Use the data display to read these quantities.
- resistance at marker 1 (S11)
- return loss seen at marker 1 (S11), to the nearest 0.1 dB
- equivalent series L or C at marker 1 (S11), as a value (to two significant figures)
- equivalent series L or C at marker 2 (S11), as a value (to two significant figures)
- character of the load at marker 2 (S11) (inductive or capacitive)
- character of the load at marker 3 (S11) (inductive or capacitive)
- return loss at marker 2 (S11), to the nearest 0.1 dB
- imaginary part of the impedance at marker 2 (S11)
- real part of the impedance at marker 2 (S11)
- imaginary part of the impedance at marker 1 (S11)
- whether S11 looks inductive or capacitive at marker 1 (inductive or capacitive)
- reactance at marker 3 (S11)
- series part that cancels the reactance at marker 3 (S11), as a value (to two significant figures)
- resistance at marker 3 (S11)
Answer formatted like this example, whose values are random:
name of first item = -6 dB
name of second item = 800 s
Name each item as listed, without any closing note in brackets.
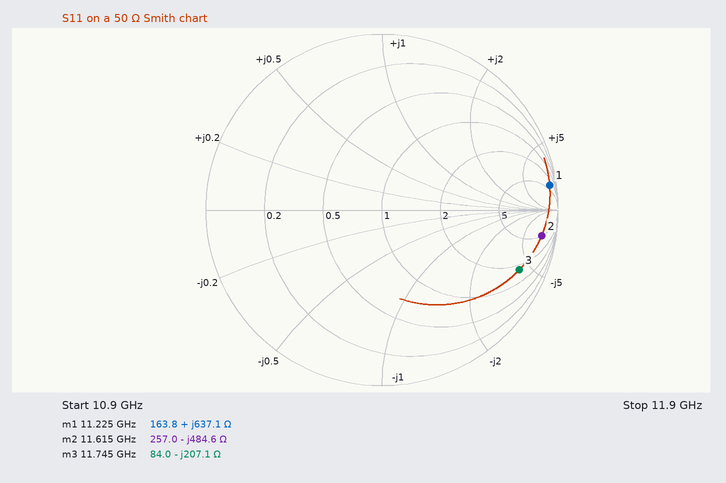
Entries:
resistance at marker 1 = 163.8 Ω
return loss seen at marker 1 (S11), to the nearest 0.1 dB = 0.3 dB
equivalent series L or C at marker 1 (S11), as a value = 9.0 nH
equivalent series L or C at marker 2 (S11), as a value = 28 fF
character of the load at marker 2 (S11) = capacitive
character of the load at marker 3 (S11) = capacitive
return loss at marker 2 (S11), to the nearest 0.1 dB = 0.7 dB
imaginary part of the impedance at marker 2 = -484.6 Ω
real part of the impedance at marker 2 = 257.0 Ω
imaginary part of the impedance at marker 1 = +637.1 Ω
whether S11 looks inductive or capacitive at marker 1 = inductive
reactance at marker 3 = -207.1 Ω
series part that cancels the reactance at marker 3 (S11), as a value = 2.8 nH
resistance at marker 3 = 84.0 Ω
